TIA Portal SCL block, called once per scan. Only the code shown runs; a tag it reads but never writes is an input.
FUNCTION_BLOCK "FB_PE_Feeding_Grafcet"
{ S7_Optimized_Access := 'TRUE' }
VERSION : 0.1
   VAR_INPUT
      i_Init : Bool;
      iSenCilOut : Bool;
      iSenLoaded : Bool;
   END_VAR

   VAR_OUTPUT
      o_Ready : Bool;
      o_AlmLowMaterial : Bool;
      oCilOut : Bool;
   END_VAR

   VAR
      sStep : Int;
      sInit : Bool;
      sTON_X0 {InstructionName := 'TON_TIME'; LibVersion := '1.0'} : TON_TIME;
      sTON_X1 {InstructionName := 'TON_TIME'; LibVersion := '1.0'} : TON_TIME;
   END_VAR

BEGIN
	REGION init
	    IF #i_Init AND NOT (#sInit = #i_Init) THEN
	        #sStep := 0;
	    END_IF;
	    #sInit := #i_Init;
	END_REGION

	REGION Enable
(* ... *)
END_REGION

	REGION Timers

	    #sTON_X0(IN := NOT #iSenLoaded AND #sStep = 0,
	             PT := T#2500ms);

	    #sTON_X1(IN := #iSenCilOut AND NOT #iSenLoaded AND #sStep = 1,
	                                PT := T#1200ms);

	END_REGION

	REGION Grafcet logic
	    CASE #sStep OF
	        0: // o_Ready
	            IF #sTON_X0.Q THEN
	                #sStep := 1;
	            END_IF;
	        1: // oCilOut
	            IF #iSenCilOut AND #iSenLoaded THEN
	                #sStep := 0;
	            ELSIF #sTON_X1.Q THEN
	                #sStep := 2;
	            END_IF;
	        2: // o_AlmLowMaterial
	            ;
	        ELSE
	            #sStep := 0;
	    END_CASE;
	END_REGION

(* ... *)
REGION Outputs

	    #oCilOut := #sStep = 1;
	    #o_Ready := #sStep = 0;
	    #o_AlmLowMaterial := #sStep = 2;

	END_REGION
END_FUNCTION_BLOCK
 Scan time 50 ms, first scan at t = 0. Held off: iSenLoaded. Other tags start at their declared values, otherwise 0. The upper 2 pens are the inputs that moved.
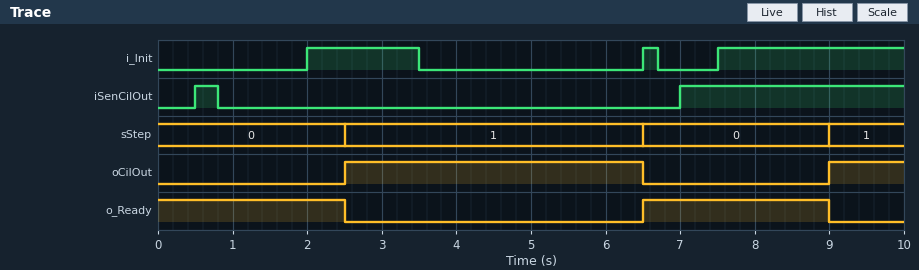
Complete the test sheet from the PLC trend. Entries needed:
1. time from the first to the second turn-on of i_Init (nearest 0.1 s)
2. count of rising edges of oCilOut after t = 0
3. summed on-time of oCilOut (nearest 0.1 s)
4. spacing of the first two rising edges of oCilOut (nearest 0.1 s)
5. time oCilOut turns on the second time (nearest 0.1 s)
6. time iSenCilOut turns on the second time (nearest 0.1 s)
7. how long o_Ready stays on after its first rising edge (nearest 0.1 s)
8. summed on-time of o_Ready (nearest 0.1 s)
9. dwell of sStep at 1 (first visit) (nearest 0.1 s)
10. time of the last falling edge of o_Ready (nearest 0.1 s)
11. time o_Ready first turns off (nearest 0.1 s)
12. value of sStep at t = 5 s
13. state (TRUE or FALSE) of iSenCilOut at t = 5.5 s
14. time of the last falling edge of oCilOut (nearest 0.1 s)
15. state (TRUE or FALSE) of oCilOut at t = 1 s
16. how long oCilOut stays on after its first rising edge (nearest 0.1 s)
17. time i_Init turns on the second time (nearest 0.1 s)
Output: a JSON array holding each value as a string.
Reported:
["4.5 s", "2", "5.0 s", "6.5 s", "9.0 s", "7.0 s", "2.5 s", "5.0 s", "4.0 s", "9.0 s", "2.5 s", "1", "FALSE", "6.5 s", "FALSE", "4.0 s", "6.5 s"]
